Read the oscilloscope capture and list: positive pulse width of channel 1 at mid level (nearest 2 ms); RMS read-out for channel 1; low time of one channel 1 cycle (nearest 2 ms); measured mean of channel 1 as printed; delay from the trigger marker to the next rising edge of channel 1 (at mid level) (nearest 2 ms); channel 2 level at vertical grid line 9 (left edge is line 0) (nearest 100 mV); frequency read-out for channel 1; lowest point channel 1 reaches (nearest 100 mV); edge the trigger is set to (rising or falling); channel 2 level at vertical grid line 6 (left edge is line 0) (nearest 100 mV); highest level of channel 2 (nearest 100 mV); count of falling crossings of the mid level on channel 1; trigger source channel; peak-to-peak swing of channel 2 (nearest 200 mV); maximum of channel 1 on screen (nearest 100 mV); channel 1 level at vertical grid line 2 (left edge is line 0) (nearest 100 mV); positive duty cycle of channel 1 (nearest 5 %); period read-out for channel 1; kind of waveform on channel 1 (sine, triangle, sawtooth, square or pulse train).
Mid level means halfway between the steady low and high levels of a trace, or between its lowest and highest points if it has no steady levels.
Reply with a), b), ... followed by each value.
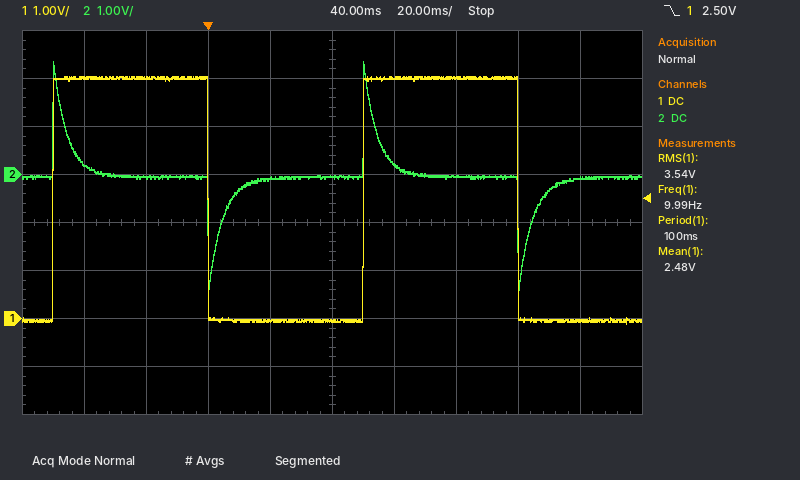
a) 50 ms
b) 3.54 V
c) 50 ms
d) 2.48 V
e) 50 ms
f) -100 mV
g) 9.99 Hz
h) -100 mV
i) falling
j) 200 mV
k) 2.4 V
l) 2
m) channel 1
n) 4.8 V
o) 5.0 V
p) 5.0 V
q) 50 %
r) 100 ms
s) square
